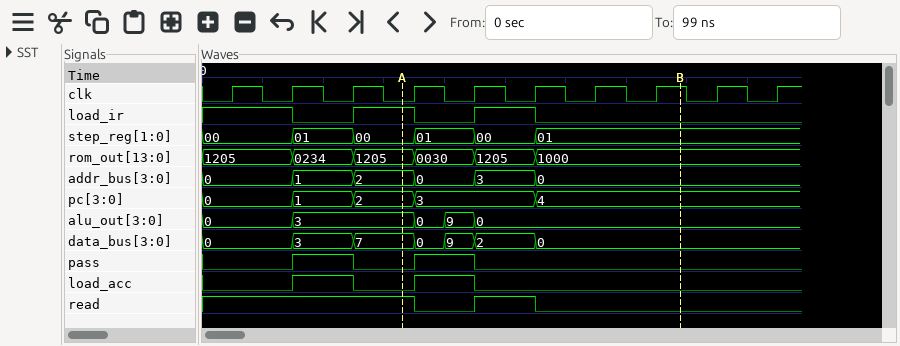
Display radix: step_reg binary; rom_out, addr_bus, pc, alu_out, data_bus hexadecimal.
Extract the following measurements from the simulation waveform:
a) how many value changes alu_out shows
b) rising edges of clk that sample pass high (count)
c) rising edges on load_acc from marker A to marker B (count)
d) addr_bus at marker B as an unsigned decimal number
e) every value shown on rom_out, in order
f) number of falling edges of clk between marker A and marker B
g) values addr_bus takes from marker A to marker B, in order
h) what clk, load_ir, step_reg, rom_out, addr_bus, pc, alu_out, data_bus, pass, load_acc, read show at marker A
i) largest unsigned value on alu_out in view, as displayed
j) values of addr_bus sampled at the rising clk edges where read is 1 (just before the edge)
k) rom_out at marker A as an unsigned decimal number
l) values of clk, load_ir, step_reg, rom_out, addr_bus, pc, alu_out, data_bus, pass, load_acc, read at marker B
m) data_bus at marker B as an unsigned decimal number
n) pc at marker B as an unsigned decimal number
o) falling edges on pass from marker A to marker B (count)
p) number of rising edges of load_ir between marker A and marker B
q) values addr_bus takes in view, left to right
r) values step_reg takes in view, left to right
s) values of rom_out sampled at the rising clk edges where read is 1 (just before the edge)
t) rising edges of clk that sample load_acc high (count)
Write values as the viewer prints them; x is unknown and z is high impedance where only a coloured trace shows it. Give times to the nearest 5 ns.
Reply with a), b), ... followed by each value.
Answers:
a) 4
b) 2
c) 1
d) 0
e) 1205, 0234, 1205, 0030, 1205, 1000
f) 4
g) 2, 0, 3, 0
h) clk=0, load_ir=1, step_reg=00, rom_out=1205, addr_bus=2, pc=2, alu_out=3, data_bus=7, pass=0, load_acc=0, read=1
i) 9
j) 0, 0, 1, 2, 3
k) 4613
l) clk=1, load_ir=0, step_reg=01, rom_out=1000, addr_bus=0, pc=4, alu_out=0, data_bus=0, pass=0, load_acc=0, read=0
m) 0
n) 4
o) 1
p) 1
q) 0, 1, 2, 0, 3, 0
r) 00, 01, 00, 01, 00, 01
s) 1205, 1205, 0234, 1205, 1205
t) 2
